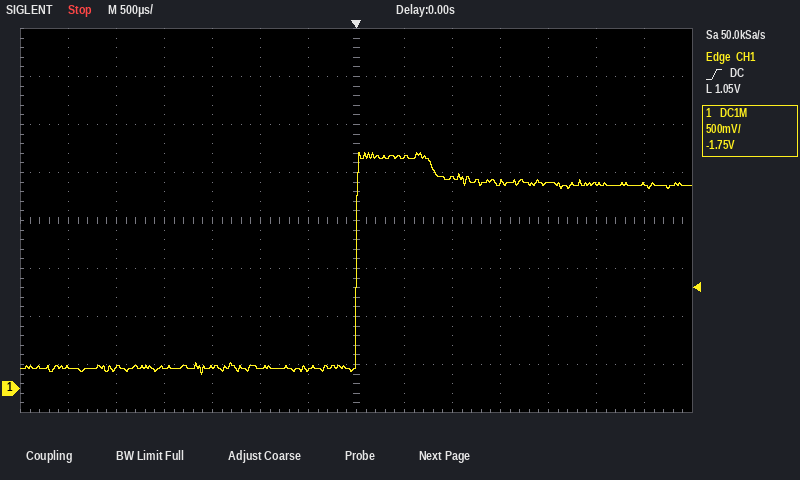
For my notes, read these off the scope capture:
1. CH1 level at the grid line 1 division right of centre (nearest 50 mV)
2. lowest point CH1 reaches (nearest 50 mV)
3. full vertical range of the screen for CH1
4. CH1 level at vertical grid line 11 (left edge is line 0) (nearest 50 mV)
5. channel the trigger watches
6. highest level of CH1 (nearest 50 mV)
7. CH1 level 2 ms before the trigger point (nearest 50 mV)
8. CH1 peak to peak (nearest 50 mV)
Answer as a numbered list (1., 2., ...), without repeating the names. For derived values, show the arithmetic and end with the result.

1. 2.40 V
2. 150 mV
3. 4 V
4. 2.15 V
5. CH1
6. 2.45 V
7. 200 mV
8. 2.45 V − (150 mV) = 2.30 V
